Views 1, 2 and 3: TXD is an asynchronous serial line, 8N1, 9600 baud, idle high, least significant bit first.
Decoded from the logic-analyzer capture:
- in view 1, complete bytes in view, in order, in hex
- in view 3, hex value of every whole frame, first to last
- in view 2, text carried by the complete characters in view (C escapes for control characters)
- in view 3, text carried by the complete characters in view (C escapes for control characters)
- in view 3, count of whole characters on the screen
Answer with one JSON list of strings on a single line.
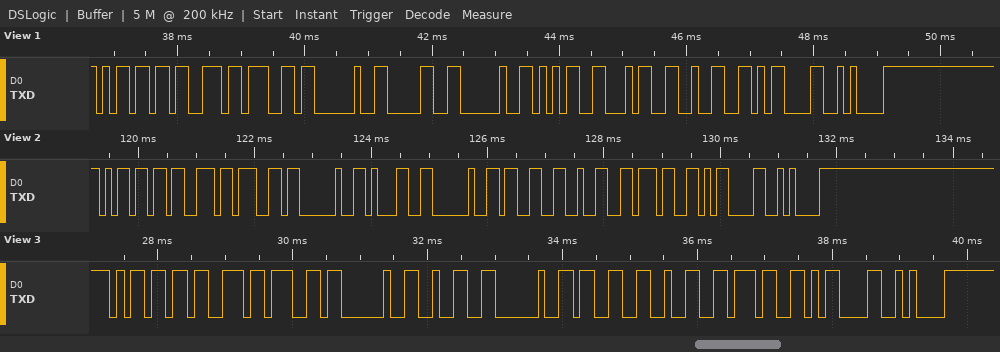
["6D 73 67 20 30 20 35 34 32 0D 0A", "0x6D 0x73 0x67 0x20 0x32 0x20 0x33 0x32 0x37 0x0D 0x0A", "\"msg 1 327\\r\\n\"", "\"msg 2 327\\r\\n\"", "11"]
